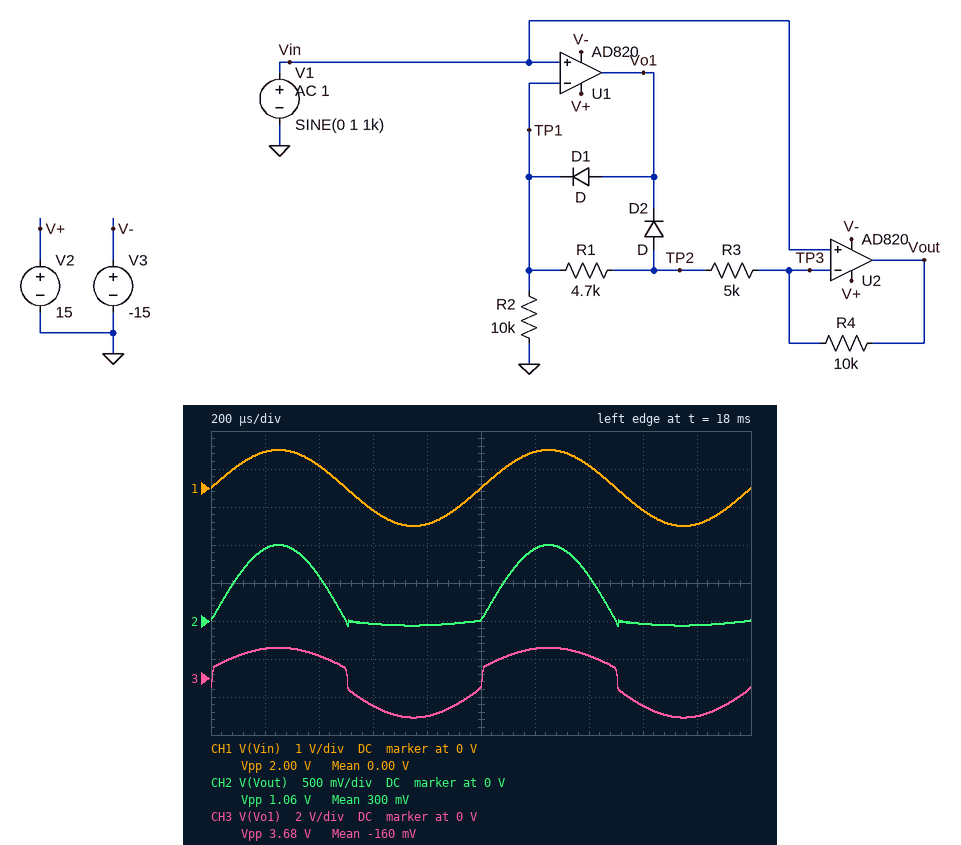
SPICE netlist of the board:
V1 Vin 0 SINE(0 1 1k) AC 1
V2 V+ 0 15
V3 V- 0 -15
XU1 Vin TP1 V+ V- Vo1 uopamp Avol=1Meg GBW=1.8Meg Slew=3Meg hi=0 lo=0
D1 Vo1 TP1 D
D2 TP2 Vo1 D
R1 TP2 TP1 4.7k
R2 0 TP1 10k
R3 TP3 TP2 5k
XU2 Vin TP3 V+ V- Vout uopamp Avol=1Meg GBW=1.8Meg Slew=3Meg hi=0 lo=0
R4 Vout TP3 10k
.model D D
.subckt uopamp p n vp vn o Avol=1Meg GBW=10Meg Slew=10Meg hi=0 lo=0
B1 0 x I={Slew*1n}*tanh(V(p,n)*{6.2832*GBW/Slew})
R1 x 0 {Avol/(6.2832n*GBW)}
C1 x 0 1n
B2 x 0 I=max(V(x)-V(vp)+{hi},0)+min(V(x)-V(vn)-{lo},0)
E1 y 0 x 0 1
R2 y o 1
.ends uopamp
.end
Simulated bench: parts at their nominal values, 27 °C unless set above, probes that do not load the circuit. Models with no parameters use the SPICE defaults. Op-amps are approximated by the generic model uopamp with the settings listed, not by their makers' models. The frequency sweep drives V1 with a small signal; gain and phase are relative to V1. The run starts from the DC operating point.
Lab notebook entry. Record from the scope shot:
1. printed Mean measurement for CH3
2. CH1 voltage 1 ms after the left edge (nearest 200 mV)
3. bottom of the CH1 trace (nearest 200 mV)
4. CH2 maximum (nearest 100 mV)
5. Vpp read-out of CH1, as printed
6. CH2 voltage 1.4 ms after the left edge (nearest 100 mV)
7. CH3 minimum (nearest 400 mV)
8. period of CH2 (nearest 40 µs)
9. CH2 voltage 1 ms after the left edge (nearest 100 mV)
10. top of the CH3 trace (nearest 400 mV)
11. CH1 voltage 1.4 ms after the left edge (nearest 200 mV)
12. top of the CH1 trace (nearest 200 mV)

-160 mV
0 V
-1.0 V
1.0 V
2.00 V
600 mV
-2.0 V
1.00 ms
0 V
1.6 V
600 mV
1.0 V
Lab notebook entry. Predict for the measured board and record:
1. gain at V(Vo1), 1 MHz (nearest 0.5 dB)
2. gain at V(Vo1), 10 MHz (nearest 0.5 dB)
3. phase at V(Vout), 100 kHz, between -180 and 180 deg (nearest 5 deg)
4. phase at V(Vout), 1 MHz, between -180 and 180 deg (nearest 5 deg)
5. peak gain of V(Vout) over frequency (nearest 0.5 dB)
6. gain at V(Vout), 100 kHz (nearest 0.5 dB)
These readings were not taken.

2.5 dB
-15.0 dB
-5 deg
-40 deg
3.5 dB
3.5 dB
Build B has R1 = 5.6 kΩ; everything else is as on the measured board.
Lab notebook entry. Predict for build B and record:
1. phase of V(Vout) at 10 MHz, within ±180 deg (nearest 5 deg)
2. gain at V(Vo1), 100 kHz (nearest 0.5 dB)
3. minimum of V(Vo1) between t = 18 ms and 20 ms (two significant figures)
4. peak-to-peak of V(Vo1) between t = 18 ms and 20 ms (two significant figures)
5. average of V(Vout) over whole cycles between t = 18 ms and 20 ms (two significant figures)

-85 deg
19.5 dB
-2.2 V
3.8 V
360 mV
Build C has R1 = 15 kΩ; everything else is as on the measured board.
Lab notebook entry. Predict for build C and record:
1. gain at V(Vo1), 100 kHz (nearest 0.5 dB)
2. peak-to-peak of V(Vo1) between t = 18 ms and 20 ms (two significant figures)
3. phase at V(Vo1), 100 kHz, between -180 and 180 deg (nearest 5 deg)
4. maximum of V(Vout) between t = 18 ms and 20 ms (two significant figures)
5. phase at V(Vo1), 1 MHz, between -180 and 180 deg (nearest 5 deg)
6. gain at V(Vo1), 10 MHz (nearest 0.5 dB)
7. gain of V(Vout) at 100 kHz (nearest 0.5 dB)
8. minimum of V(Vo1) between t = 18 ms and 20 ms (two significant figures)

21.5 dB
4.7 V
-90 deg
2.0 V
-80 deg
-15.0 dB
2.5 dB
-3.1 V
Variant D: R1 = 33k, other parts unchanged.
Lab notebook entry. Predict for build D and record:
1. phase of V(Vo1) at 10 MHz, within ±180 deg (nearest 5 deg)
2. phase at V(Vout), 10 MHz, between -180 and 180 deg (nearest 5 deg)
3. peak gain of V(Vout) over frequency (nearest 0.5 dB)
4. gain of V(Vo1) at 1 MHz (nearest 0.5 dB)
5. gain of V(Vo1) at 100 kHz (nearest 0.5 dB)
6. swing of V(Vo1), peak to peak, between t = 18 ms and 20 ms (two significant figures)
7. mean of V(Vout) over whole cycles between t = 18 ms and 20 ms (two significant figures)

-90 deg
-80 deg
1.5 dB
4.0 dB
23.0 dB
6.5 V
2.1 V
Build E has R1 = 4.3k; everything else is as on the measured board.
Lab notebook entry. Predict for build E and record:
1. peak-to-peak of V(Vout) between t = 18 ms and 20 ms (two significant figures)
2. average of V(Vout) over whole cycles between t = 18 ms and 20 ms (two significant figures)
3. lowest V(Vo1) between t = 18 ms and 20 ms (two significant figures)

1.1 V
270 mV
-2.0 V
